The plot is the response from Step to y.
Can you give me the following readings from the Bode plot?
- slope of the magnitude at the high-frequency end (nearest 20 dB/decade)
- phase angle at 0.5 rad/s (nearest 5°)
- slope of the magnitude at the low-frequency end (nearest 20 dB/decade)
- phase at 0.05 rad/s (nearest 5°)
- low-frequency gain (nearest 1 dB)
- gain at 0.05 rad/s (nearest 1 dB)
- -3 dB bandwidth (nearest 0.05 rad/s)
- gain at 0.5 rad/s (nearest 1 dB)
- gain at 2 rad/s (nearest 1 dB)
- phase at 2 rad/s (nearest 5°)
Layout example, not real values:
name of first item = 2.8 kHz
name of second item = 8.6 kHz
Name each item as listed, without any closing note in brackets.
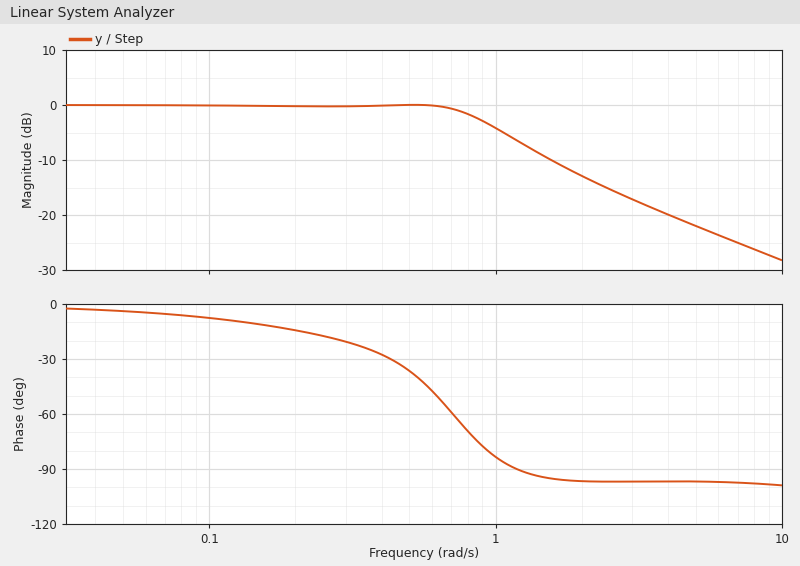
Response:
slope of the magnitude at the high-frequency end = -20 dB/decade
phase angle at 0.5 rad/s = -35°
slope of the magnitude at the low-frequency end = 0 dB/decade
phase at 0.05 rad/s = -5°
low-frequency gain = 0 dB
gain at 0.05 rad/s = 0 dB
-3 dB bandwidth = 0.90 rad/s
gain at 0.5 rad/s = 0 dB
gain at 2 rad/s = -13 dB
phase at 2 rad/s = -95°
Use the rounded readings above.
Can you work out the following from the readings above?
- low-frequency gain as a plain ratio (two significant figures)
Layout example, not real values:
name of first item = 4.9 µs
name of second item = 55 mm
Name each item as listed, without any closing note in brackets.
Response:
low-frequency gain as a plain ratio = 1.0
